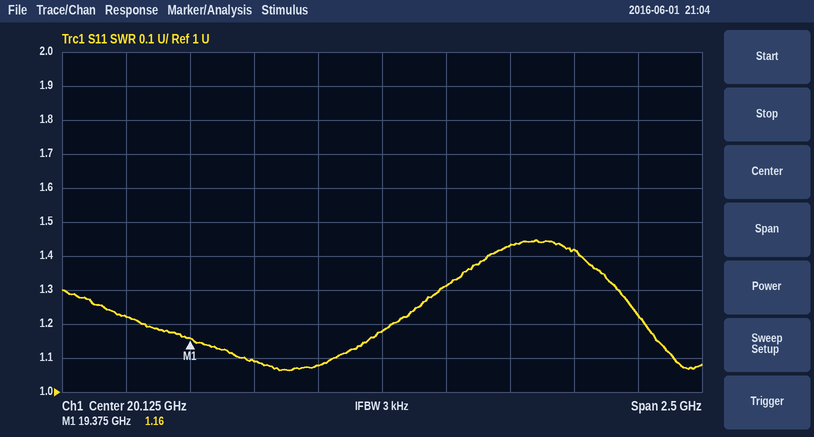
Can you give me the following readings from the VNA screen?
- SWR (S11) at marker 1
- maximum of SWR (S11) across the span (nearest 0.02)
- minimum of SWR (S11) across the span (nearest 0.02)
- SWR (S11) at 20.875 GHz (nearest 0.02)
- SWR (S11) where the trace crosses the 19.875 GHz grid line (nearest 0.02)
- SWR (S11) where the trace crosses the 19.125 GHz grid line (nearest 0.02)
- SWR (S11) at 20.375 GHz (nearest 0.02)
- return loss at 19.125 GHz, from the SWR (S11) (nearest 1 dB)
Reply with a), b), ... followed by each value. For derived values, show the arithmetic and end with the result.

a) 1.16
b) 1.44
c) 1.06
d) 1.42
e) 1.08
f) 1.22
g) 1.32
h) −20 log10((1.22 − 1)/(1.22 + 1)) ≈ 20 dB
